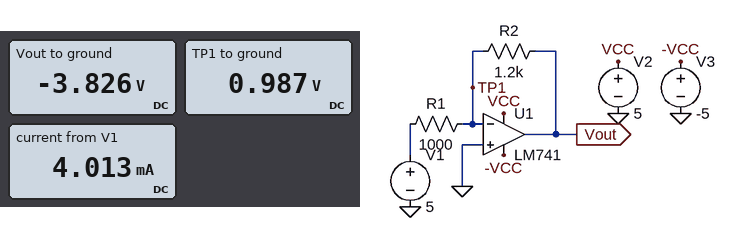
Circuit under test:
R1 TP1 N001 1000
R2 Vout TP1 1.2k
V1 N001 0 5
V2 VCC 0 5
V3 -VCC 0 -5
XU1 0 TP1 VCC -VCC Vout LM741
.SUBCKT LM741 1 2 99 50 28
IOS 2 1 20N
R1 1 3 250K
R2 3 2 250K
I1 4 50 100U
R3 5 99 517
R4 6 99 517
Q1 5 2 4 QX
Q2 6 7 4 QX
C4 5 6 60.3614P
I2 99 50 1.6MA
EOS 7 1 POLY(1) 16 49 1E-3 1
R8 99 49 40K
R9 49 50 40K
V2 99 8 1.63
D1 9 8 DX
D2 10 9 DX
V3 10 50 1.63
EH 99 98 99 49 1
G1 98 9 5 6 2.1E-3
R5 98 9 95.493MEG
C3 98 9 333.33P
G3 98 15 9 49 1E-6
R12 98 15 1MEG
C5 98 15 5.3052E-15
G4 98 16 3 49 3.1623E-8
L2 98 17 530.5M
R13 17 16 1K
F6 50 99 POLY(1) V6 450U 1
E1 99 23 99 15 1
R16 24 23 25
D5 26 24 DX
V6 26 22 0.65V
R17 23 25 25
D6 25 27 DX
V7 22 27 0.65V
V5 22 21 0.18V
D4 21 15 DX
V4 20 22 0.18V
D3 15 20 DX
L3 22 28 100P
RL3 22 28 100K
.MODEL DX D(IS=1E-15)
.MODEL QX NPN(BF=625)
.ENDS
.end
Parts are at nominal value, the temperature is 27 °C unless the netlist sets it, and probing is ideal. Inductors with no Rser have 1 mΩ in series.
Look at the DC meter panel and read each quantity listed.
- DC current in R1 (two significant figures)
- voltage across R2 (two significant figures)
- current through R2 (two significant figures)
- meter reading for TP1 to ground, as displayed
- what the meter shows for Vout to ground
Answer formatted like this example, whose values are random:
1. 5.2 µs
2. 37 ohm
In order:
1. 4.0 mA
2. 4.8 V
3. 4.0 mA
4. 0.987 V
5. -3.826 V
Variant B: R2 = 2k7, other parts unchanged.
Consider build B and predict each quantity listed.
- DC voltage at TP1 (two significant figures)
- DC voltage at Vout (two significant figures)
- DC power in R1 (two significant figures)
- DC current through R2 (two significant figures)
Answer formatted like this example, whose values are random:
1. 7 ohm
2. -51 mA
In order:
1. 2.6 V
2. -3.9 V
3. 5.8 mW
4. 2.4 mA
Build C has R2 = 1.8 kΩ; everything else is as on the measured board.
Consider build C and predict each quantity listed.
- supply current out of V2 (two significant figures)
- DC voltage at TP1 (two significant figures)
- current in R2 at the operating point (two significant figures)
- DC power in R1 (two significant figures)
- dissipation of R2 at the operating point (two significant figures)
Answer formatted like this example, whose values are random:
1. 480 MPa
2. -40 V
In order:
1. 1.3 mA
2. 1.8 V
3. 3.2 mA
4. 10 mW
5. 18 mW
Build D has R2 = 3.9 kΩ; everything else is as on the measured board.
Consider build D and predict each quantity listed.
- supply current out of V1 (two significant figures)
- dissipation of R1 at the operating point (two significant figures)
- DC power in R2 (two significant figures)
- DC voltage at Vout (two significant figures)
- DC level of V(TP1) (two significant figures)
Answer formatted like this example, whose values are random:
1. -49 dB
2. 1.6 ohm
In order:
1. 1.8 mA
2. 3.3 mW
3. 13 mW
4. -3.9 V
5. 3.2 V
